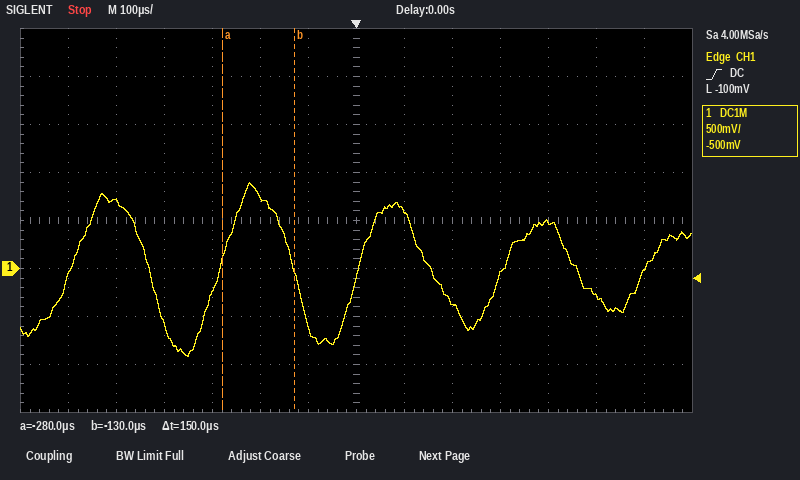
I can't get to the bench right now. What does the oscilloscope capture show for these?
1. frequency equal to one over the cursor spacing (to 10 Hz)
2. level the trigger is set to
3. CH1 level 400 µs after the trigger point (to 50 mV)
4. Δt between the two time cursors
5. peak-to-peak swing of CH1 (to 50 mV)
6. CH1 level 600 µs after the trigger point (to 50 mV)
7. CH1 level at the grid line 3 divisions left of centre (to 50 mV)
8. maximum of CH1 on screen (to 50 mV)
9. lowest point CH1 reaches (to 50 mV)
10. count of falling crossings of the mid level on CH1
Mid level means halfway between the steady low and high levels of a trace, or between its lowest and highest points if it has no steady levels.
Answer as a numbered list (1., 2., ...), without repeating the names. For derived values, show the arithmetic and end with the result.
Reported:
1. 1 / 150 µs ≈ 6.67 kHz
2. -100 mV
3. 500 mV
4. 150 µs
5. 900 mV − (-900 mV) = 1.80 V
6. 0 mV
7. -250 mV
8. 900 mV
9. -900 mV
10. 4
